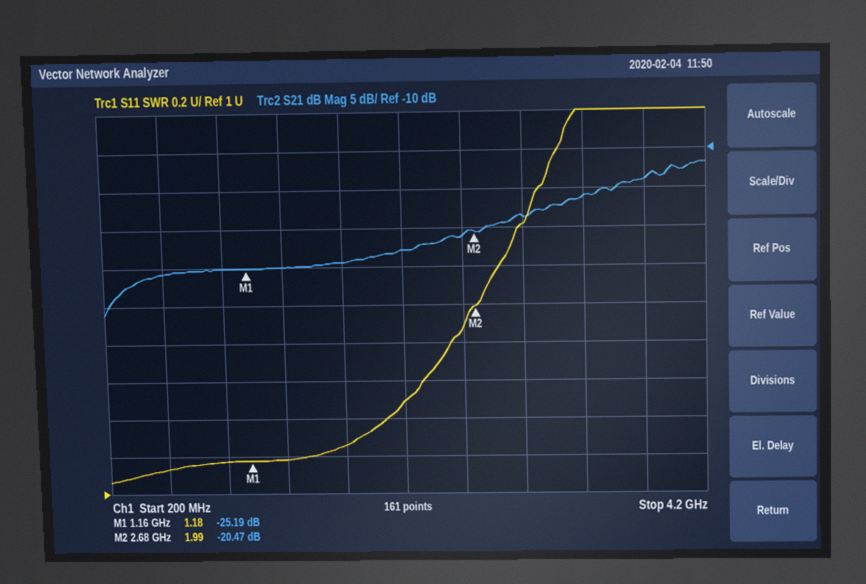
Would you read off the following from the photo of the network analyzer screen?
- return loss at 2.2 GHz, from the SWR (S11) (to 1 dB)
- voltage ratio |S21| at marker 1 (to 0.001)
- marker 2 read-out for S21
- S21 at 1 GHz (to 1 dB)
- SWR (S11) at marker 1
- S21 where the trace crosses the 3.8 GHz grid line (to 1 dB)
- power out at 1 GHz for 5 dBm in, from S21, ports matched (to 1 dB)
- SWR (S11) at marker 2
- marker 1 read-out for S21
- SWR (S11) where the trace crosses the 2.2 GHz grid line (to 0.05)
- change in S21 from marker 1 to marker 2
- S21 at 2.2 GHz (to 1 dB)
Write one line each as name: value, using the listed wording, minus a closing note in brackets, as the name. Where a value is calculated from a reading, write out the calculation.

return loss at 2.2 GHz, from the SWR (S11): −20 log10((1.5 − 1)/(1.5 + 1)) ≈ 14 dB
voltage ratio |S21| at marker 1: 10^(-25.19/20) ≈ 0.055
marker 2 read-out for S21: -20.47 dB
S21 at 1 GHz: -25 dB
SWR (S11) at marker 1: 1.18
S21 where the trace crosses the 3.8 GHz grid line: -14 dB
power out at 1 GHz for 5 dBm in, from S21, ports matched: 5 dBm + (-25 dB) = -20 dBm
SWR (S11) at marker 2: 1.99
marker 1 read-out for S21: -25.19 dB
SWR (S11) where the trace crosses the 2.2 GHz grid line: 1.50
change in S21 from marker 1 to marker 2: -20.47 − (-25.19) = 4.72 dB
S21 at 2.2 GHz: -23 dB
